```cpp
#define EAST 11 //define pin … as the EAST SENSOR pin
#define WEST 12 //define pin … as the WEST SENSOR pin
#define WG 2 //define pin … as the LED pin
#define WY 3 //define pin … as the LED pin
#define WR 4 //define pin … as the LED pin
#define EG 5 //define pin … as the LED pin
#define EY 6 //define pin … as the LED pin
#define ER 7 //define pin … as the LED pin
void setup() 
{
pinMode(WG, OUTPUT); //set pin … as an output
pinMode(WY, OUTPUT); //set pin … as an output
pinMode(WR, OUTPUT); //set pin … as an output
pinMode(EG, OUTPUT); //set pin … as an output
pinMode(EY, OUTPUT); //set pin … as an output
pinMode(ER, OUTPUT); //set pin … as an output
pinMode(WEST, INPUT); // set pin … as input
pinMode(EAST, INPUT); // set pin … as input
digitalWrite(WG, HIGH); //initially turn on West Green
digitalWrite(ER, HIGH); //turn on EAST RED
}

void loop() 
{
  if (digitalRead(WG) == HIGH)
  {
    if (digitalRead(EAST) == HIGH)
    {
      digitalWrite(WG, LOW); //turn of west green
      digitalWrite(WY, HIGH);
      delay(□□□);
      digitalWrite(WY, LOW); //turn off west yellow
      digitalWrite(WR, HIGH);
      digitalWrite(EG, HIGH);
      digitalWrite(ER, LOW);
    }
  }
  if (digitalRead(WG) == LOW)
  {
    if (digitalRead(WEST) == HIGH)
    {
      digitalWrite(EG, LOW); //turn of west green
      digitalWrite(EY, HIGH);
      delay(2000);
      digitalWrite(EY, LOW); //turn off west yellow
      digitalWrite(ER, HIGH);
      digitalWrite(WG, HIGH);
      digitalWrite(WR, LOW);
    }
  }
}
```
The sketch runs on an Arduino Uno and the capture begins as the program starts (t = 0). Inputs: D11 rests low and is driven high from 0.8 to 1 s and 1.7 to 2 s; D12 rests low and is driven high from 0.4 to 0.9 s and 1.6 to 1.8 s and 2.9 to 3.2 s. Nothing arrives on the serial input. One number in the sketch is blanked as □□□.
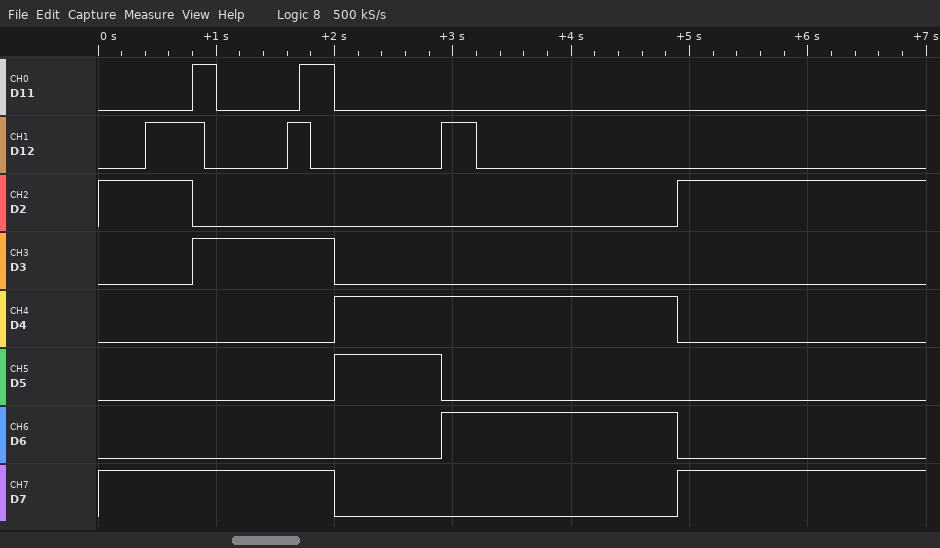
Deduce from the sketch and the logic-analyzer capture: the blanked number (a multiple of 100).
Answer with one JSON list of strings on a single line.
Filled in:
["1200"]
